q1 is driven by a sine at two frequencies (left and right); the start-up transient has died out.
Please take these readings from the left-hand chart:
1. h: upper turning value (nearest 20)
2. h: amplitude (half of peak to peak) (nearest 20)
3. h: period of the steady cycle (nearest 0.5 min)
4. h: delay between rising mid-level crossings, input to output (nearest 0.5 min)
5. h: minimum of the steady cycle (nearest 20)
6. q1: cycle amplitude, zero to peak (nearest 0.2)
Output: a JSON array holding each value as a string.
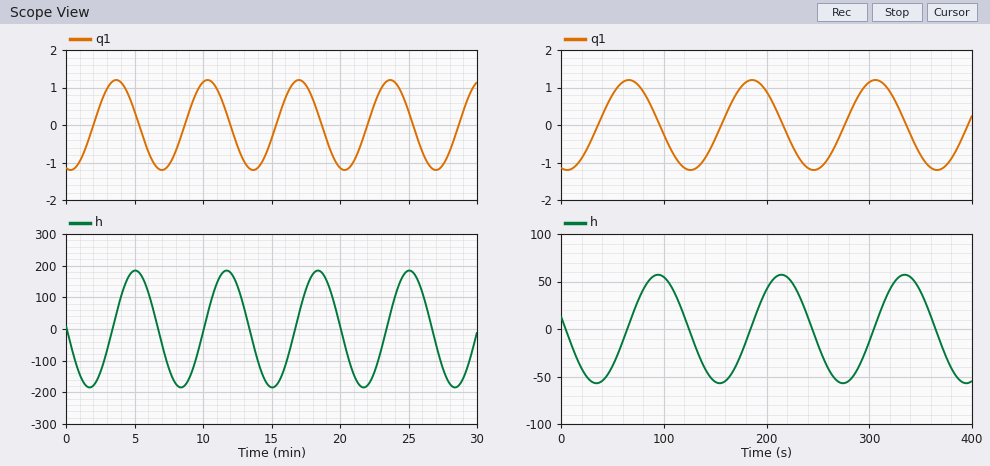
["180", "180", "6.5 min", "1.5 min", "-180", "1.2"]
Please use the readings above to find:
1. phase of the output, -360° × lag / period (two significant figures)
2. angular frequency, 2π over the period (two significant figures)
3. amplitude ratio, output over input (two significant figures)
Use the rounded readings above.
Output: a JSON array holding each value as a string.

["-83°", "0.97 rad/min", "150"]
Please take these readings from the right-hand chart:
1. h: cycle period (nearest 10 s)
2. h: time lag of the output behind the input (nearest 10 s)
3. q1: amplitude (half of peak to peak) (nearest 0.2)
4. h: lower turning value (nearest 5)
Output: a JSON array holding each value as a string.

["120 s", "30 s", "1.2", "-55"]
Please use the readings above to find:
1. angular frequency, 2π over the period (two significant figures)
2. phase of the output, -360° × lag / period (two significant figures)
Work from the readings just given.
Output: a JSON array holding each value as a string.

["0.052 rad/s", "-90°"]
